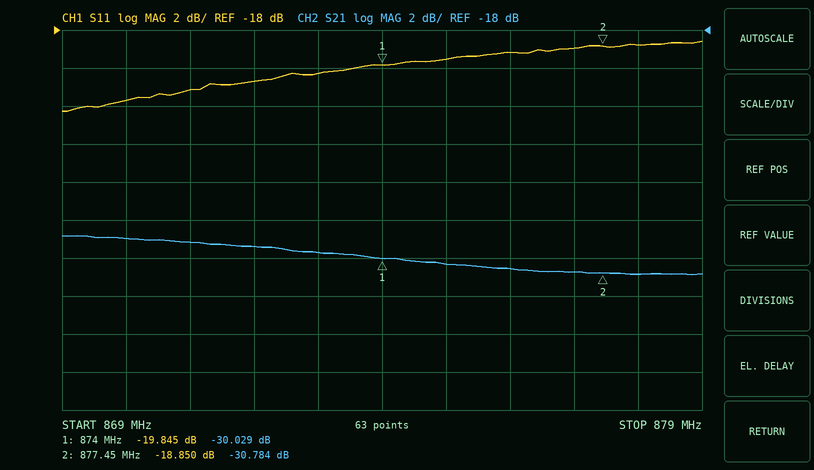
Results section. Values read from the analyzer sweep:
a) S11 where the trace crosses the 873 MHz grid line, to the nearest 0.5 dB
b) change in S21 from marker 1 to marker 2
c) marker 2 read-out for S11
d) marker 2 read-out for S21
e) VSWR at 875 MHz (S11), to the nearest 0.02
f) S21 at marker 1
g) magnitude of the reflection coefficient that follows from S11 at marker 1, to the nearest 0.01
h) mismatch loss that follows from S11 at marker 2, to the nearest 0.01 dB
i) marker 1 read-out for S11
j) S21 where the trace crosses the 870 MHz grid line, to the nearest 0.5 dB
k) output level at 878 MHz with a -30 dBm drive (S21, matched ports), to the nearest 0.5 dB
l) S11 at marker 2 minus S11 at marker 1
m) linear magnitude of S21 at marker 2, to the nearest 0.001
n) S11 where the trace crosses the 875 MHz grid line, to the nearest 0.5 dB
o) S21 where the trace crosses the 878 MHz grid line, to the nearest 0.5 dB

-20.5 dB
-0.755 dB
-18.850 dB
-30.784 dB
1.24
-30.029 dB
0.10
0.06 dB
-19.845 dB
-29.0 dB
-61.0 dBm
0.995 dB
0.029
-19.5 dB
-31.0 dB
